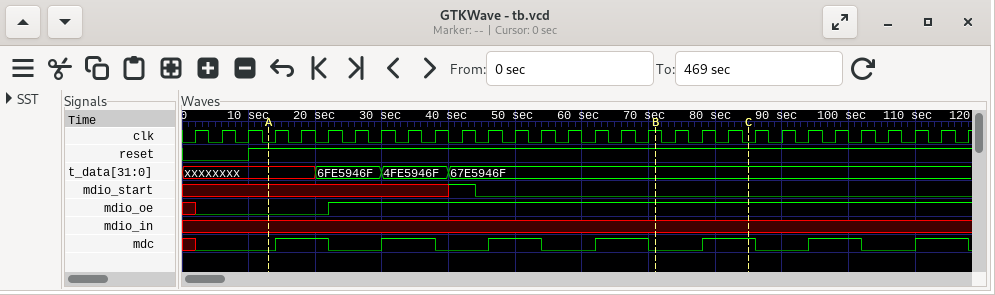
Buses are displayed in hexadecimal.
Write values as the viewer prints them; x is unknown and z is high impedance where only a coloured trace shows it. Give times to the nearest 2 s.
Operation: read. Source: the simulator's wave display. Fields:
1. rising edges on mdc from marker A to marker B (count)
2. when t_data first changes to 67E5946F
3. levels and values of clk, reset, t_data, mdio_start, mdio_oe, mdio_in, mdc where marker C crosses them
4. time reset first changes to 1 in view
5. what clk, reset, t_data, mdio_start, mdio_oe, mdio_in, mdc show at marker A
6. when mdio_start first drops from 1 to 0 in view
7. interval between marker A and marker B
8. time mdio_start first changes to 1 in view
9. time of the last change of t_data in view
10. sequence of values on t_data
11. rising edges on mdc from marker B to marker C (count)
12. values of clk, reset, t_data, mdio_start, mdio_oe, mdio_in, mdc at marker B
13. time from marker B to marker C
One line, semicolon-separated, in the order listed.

4; 40 s; clk=0, reset=1, t_data=67E5946F, mdio_start=0, mdio_oe=1, mdio_in=x, mdc=1; 10 s; clk=0, reset=1, t_data=xxxxxxxx, mdio_start=x, mdio_oe=0, mdio_in=x, mdc=0; 44 s; 58 s; 40 s; 40 s; xxxxxxxx, 6FE5946F, 4FE5946F, 67E5946F; 1; clk=1, reset=1, t_data=67E5946F, mdio_start=0, mdio_oe=1, mdio_in=x, mdc=0; 14 s
